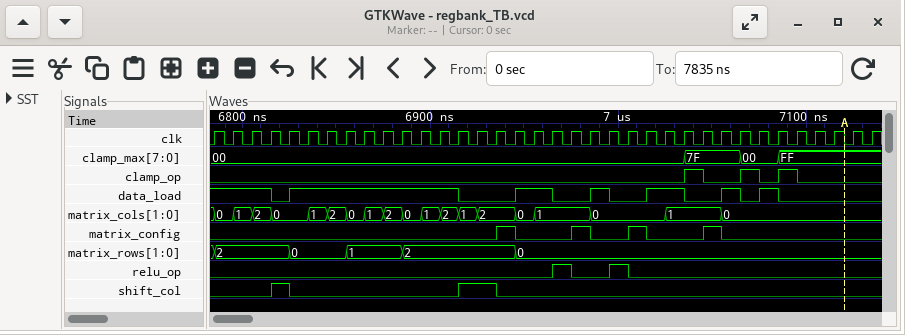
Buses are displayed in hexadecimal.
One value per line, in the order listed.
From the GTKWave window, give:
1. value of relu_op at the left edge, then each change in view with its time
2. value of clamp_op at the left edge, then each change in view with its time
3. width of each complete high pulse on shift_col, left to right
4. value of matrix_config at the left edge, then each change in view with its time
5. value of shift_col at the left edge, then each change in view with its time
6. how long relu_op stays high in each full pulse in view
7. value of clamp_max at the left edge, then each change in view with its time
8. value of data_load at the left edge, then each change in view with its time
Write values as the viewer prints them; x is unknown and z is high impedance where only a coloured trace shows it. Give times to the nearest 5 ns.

0, 1 at 6965 ns, 0 at 6975 ns, 1 at 6995 ns, 0 at 7005 ns
0, 1 at 7035 ns, 0 at 7045 ns, 1 at 7065 ns, 0 at 7075 ns, 1 at 7085 ns, 0 at 7095 ns
10 ns, 20 ns
0, 1 at 6935 ns, 0 at 6945 ns, 1 at 6975 ns, 0 at 6985 ns, 1 at 7005 ns, 0 at 7015 ns, 1 at 7045 ns, 0 at 7055 ns
0, 1 at 6815 ns, 0 at 6825 ns, 1 at 6915 ns, 0 at 6935 ns
10 ns, 10 ns
00, 7F at 7035 ns, 00 at 7065 ns, FF at 7085 ns
1, 0 at 6815 ns, 1 at 6825 ns, 0 at 6915 ns, 1 at 6945 ns, 0 at 6965 ns, 1 at 6985 ns, 0 at 6995 ns, 1 at 7015 ns, 0 at 7035 ns, 1 at 7055 ns, 0 at 7065 ns, 1 at 7075 ns, 0 at 7085 ns
